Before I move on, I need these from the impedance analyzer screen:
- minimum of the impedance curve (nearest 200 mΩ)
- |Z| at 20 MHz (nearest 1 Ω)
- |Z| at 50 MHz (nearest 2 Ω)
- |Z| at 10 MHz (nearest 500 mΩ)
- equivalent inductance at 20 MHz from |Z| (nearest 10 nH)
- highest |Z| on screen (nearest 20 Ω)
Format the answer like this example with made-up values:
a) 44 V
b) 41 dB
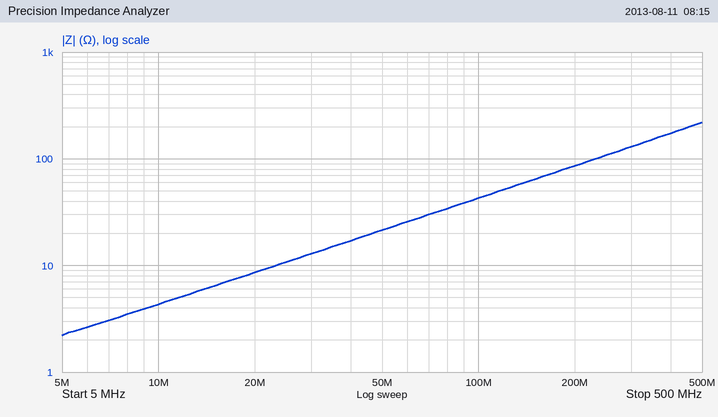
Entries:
a) 2.2 Ω
b) 9 Ω
c) 22 Ω
d) 4.5 Ω
e) 70 nH
f) 220 Ω
